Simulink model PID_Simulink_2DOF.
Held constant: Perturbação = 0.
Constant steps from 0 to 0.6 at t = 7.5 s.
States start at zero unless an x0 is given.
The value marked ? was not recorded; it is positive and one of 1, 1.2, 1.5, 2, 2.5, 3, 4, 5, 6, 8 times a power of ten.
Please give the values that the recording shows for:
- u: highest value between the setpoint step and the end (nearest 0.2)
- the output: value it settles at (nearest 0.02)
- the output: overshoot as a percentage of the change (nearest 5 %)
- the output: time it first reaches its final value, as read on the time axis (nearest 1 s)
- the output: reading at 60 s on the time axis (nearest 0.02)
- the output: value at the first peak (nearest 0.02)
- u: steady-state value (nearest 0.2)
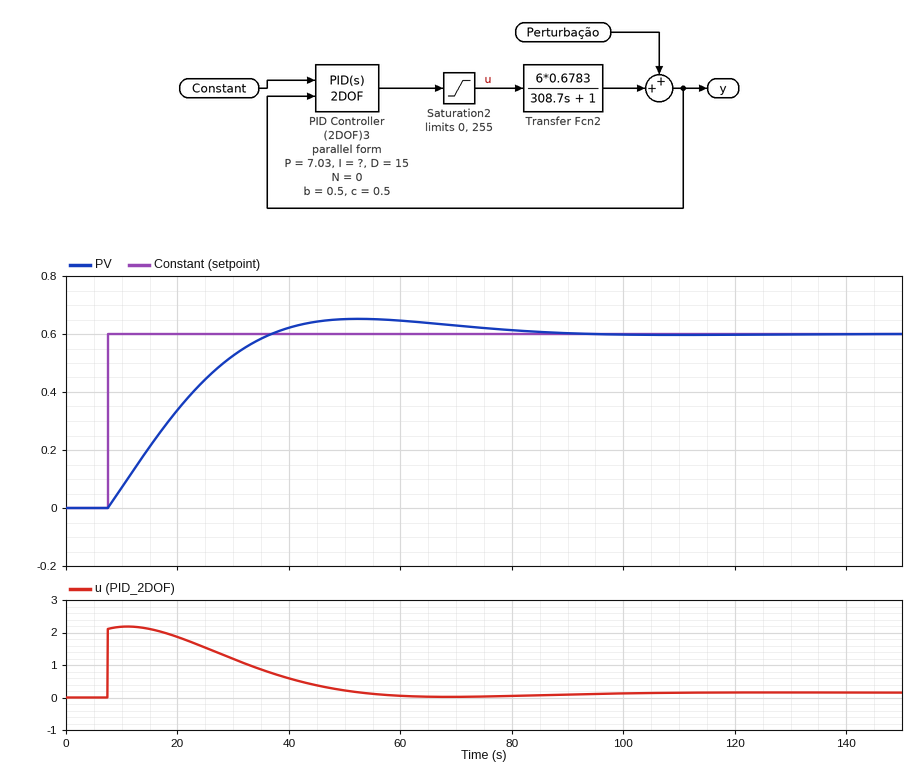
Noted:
2.2
0.60
10 %
37 s
0.64
0.66
0.2
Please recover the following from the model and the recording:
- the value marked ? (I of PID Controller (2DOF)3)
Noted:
0.4
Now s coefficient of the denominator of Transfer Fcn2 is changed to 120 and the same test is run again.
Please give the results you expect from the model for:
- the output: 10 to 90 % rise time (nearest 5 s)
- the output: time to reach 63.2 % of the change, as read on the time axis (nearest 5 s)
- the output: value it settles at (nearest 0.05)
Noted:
20 s
15 s
0.60
